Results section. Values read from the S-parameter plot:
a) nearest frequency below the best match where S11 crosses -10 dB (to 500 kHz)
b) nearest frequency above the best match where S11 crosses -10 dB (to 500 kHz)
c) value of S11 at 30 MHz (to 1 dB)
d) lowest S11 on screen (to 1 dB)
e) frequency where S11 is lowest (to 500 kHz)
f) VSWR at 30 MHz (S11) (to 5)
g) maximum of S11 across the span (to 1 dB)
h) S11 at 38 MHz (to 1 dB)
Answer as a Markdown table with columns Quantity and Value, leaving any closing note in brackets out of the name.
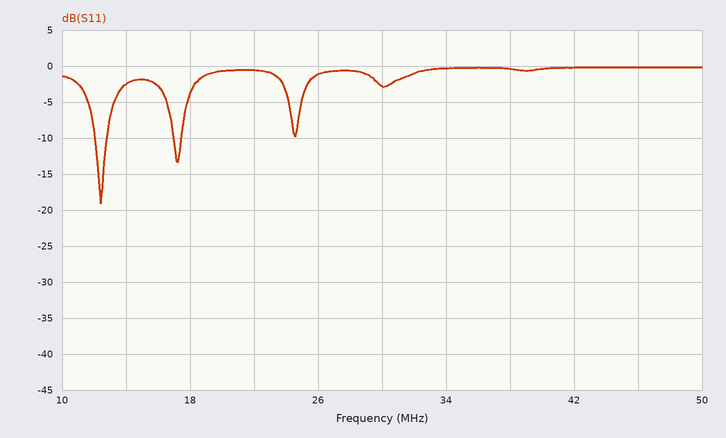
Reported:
| Quantity | Value |
|---|---|
| nearest frequency below the best match where S11 crosses -10 dB | 12.0 MHz |
| nearest frequency above the best match where S11 crosses -10 dB | 13.0 MHz |
| value of S11 at 30 MHz | -3 dB |
| lowest S11 on screen | -19 dB |
| frequency where S11 is lowest | 12.5 MHz |
| VSWR at 30 MHz (S11) | 5 |
| maximum of S11 across the span | 0 dB |
| S11 at 38 MHz | 0 dB |
